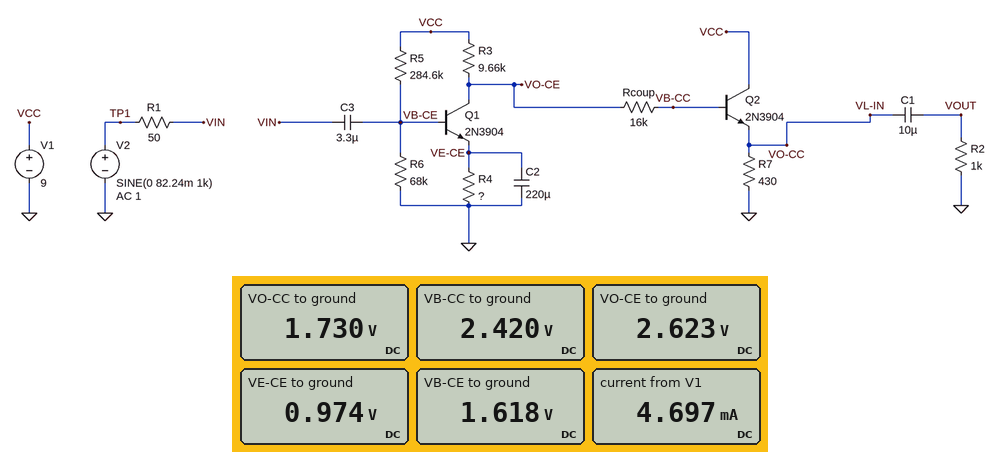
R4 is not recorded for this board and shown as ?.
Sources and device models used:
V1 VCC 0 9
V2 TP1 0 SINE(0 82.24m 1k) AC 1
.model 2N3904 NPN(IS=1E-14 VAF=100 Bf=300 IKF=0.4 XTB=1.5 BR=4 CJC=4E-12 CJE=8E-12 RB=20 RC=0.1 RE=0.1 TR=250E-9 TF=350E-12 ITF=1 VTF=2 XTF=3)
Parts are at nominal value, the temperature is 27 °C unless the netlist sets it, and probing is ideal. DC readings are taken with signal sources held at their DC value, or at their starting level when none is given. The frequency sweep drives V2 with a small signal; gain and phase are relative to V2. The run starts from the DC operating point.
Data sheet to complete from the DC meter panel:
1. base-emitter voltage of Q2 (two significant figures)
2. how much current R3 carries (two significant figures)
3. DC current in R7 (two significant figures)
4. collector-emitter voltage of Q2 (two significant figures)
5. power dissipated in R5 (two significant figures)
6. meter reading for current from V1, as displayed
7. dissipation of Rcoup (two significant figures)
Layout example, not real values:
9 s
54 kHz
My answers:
690 mV
660 µA
4.0 mA
7.3 V
190 µW
4.697 mA
2.6 µW
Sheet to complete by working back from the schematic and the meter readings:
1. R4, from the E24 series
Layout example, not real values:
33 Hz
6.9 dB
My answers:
1.5 kΩ
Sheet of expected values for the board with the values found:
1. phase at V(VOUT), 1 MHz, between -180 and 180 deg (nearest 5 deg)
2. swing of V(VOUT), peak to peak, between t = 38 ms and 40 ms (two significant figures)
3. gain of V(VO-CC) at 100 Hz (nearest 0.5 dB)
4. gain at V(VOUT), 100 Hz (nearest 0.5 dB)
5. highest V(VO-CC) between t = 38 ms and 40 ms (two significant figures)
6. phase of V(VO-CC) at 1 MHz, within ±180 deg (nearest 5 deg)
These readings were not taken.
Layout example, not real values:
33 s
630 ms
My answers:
135 deg
5.3 V
44.5 dB
44.5 dB
6.7 V
135 deg
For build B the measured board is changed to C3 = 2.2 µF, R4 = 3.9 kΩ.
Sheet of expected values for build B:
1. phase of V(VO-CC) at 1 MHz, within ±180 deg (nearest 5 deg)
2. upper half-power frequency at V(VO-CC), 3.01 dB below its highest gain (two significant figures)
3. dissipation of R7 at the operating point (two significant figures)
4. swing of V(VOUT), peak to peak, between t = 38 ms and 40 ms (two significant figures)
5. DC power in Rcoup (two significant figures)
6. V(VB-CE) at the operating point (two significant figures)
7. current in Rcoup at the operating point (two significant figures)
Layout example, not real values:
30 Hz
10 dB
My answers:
145 deg
1.8 MHz
52 mW
5.2 V
21 µW
1.7 V
36 µA
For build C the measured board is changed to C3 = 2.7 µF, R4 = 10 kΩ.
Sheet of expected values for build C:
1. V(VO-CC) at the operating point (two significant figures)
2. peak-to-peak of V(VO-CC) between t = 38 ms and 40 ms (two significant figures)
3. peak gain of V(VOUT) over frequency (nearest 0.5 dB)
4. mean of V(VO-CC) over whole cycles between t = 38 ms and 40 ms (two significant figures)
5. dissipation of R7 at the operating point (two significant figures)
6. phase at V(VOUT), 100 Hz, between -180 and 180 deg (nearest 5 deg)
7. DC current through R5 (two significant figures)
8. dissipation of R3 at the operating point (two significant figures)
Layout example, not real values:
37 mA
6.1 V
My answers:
6.0 V
4.9 V
30.0 dB
5.6 V
84 mW
-170 deg
26 µA
240 µW
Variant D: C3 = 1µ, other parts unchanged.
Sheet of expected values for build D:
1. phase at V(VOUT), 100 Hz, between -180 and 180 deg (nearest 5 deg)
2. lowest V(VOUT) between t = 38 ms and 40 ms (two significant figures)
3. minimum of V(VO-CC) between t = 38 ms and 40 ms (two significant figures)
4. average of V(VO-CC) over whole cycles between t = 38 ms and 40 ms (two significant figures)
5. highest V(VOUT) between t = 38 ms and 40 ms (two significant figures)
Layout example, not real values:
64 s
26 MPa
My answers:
-155 deg
-3.5 V
1.5 V
5.0 V
1.8 V
